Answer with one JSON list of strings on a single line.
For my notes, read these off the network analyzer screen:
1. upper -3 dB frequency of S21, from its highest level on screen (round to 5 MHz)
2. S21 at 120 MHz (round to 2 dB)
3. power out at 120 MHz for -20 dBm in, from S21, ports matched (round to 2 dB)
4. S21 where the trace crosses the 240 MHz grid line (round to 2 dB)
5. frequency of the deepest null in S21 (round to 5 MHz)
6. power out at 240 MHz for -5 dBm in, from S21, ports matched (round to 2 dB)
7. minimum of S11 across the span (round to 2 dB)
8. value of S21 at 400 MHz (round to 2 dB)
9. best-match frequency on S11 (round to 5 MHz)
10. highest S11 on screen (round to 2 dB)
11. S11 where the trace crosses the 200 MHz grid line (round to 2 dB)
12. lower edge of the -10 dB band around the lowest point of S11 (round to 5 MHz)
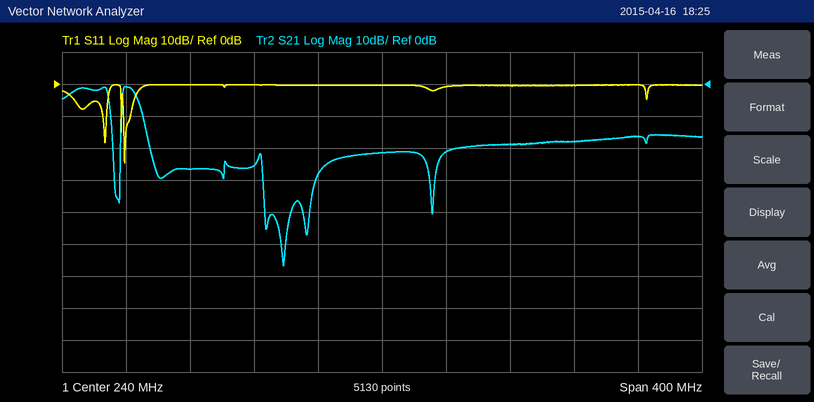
["85 MHz", "-26 dB", "-46 dBm", "-22 dB", "180 MHz", "-26 dBm", "-24 dB", "-16 dB", "80 MHz", "0 dB", "0 dB", "80 MHz"]
